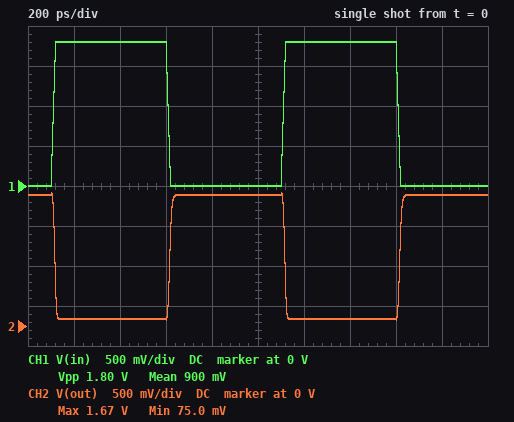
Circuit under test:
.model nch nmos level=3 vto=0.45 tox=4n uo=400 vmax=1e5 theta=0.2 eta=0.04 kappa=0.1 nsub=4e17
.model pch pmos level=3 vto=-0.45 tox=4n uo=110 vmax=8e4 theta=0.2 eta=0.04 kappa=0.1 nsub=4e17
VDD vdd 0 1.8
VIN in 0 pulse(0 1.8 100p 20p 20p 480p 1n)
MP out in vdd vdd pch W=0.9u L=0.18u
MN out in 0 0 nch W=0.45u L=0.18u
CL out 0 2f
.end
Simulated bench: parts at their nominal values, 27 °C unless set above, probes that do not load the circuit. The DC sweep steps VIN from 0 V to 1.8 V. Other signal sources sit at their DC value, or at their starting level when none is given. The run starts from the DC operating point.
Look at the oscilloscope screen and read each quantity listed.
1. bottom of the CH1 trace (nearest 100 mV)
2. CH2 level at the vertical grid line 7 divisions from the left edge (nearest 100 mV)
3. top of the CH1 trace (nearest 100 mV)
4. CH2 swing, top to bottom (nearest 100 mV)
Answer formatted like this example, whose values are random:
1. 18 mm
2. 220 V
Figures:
1. 0 V
2. 100 mV
3. 1.8 V
4. 1.6 V
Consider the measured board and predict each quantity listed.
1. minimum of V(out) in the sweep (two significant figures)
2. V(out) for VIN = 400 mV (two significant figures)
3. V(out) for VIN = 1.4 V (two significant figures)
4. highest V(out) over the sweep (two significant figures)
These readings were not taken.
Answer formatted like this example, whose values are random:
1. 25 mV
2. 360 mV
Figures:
1. 82 mV
2. 1.4 V
3. 250 mV
4. 1.6 V
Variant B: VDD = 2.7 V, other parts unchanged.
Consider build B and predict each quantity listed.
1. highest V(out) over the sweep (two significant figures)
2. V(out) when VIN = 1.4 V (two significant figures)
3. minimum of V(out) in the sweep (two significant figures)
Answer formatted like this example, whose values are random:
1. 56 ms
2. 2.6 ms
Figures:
1. 2.4 V
2. 1.3 V
3. 740 mV
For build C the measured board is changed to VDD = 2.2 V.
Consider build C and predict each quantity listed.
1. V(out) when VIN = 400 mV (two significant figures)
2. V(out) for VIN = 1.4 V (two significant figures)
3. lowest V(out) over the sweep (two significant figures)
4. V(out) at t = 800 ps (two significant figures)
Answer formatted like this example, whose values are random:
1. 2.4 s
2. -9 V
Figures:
1. 1.8 V
2. 640 mV
3. 270 mV
4. 2.0 V
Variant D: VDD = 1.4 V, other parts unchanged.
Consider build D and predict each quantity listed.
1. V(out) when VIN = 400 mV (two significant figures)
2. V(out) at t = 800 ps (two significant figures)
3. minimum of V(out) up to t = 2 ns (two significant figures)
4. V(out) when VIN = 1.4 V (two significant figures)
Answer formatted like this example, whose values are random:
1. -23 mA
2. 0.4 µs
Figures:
1. 1.0 V
2. 1.3 V
3. -17 mV
4. 48 mV
